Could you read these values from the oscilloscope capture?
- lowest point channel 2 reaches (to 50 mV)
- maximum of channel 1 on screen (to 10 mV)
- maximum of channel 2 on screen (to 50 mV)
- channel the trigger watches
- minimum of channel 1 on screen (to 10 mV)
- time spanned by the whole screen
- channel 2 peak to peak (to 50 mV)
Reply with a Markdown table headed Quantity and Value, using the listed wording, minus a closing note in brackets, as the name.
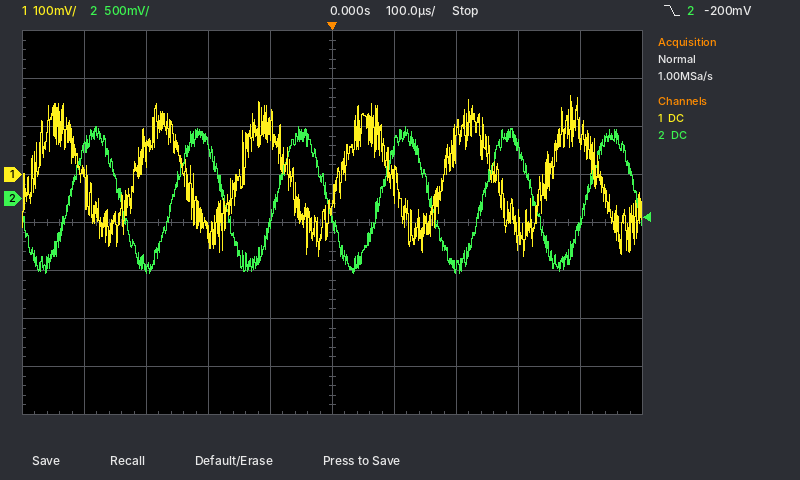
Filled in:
| Quantity | Value |
|---|---|
| lowest point channel 2 reaches | -800 mV |
| maximum of channel 1 on screen | 160 mV |
| maximum of channel 2 on screen | 750 mV |
| channel the trigger watches | channel 2 |
| minimum of channel 1 on screen | -170 mV |
| time spanned by the whole screen | 1 ms |
| channel 2 peak to peak | 1.55 V |
